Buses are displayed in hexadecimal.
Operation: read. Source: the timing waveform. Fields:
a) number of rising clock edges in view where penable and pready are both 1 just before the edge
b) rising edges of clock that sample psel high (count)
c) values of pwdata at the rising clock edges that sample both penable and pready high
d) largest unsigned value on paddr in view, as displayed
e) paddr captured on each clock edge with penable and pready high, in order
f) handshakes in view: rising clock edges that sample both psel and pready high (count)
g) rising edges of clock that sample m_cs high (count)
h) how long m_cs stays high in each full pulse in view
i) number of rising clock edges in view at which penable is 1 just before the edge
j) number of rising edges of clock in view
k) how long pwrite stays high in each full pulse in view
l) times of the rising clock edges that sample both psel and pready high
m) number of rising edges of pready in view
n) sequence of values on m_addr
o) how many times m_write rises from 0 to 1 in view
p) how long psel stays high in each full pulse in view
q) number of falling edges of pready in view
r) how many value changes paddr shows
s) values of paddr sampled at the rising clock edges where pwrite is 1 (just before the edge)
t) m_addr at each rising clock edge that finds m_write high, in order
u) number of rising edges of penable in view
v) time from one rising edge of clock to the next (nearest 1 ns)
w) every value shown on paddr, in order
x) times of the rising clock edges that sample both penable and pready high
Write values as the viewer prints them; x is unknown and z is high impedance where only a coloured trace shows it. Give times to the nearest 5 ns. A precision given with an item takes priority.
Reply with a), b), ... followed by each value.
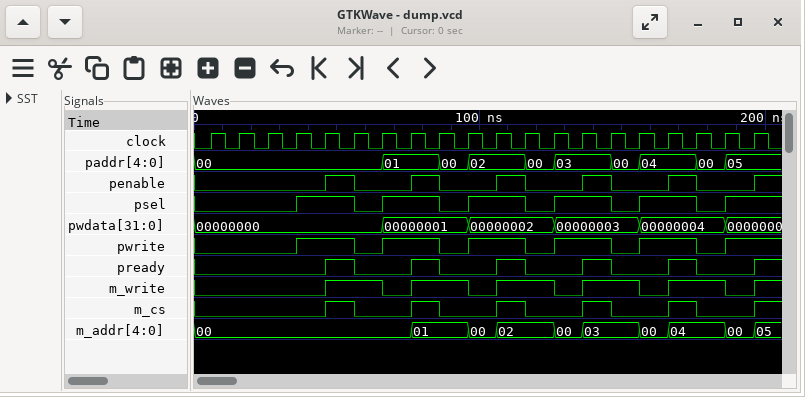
a) 5
b) 11
c) 00000000, 00000001, 00000002, 00000003, 00000004
d) 05
e) 00, 01, 02, 03, 04
f) 5
g) 5
h) 10 ns, 10 ns, 10 ns, 10 ns, 10 ns
i) 5
j) 20
k) 20 ns, 20 ns, 20 ns, 20 ns, 20 ns
l) 55 ns, 85 ns, 115 ns, 145 ns, 175 ns
m) 6
n) 00, 01, 00, 02, 00, 03, 00, 04, 00, 05
o) 6
p) 20 ns, 20 ns, 20 ns, 20 ns, 20 ns
q) 5
r) 9
s) 00, 00, 01, 01, 02, 02, 03, 03, 04, 04, 05
t) 00, 00, 01, 01, 02, 02, 03, 03, 04, 04
u) 6
v) 10 ns
w) 00, 01, 00, 02, 00, 03, 00, 04, 00, 05
x) 55 ns, 85 ns, 115 ns, 145 ns, 175 ns
